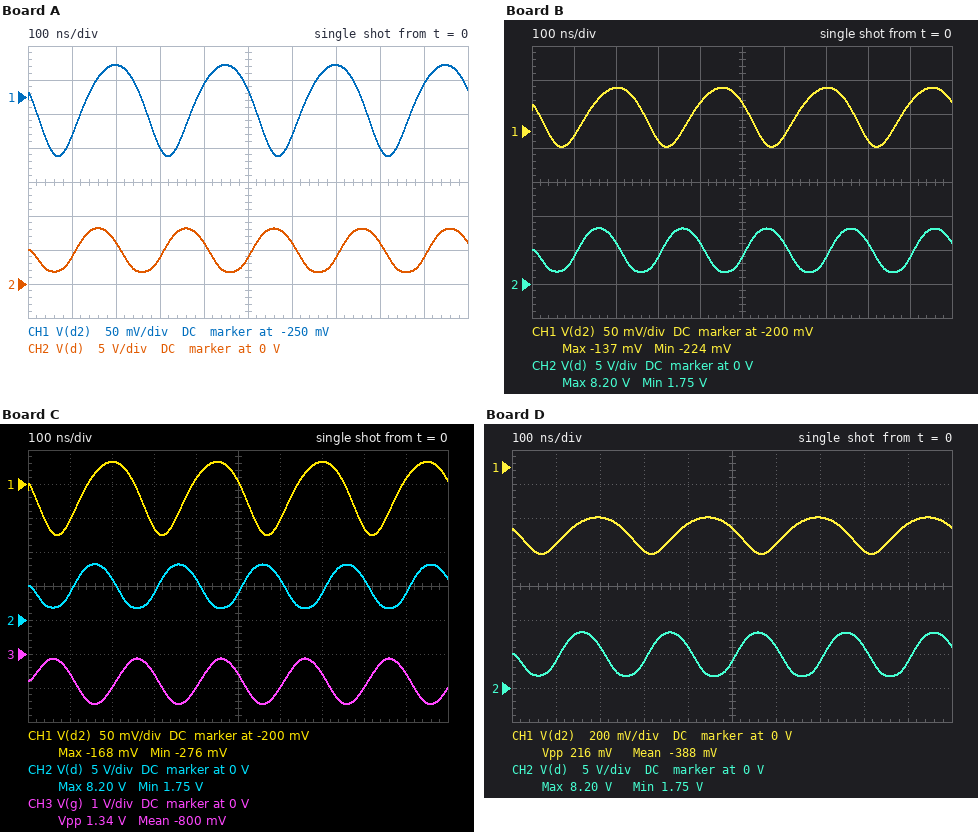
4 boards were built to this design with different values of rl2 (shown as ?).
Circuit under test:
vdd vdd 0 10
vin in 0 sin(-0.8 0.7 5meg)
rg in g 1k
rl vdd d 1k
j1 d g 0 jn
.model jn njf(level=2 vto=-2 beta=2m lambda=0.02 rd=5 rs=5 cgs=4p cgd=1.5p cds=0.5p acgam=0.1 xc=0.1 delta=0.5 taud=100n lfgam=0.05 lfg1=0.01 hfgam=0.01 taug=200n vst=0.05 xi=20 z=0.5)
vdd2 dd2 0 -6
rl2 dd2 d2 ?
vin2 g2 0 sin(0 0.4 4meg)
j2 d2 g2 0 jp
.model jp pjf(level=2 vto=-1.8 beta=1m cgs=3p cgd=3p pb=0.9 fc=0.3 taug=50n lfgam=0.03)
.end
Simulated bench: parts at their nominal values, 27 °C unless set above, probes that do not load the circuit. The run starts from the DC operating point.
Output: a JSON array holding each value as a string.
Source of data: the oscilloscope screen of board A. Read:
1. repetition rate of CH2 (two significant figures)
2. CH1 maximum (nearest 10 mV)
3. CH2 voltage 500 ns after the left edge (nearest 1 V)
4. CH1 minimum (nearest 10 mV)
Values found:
["5.0 MHz", "-200 mV", "4 V", "-340 mV"]
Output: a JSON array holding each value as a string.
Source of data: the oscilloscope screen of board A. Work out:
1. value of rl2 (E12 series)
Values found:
["6.8 kΩ"]
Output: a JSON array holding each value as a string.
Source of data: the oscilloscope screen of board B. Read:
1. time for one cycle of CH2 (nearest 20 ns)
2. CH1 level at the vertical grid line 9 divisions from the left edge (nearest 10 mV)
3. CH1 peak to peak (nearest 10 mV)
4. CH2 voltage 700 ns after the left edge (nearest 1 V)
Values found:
["200 ns", "-160 mV", "90 mV", "4 V"]
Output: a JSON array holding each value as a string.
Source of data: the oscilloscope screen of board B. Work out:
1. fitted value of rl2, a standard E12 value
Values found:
["10 kΩ"]
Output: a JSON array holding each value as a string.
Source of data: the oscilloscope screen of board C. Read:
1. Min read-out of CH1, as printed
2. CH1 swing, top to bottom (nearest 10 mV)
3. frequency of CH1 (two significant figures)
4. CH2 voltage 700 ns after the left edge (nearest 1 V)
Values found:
["-276 mV", "110 mV", "4.0 MHz", "4 V"]
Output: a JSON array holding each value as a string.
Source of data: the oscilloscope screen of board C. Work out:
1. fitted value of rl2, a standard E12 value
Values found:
["8.2 kΩ"]
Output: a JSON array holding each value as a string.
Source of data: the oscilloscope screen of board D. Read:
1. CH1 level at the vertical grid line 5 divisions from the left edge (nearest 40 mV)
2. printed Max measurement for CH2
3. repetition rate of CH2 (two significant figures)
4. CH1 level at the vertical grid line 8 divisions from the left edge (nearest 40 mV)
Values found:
["-360 mV", "8.20 V", "5.0 MHz", "-480 mV"]
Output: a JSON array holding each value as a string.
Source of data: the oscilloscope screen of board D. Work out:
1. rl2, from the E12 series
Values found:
["4.7 kΩ"]
